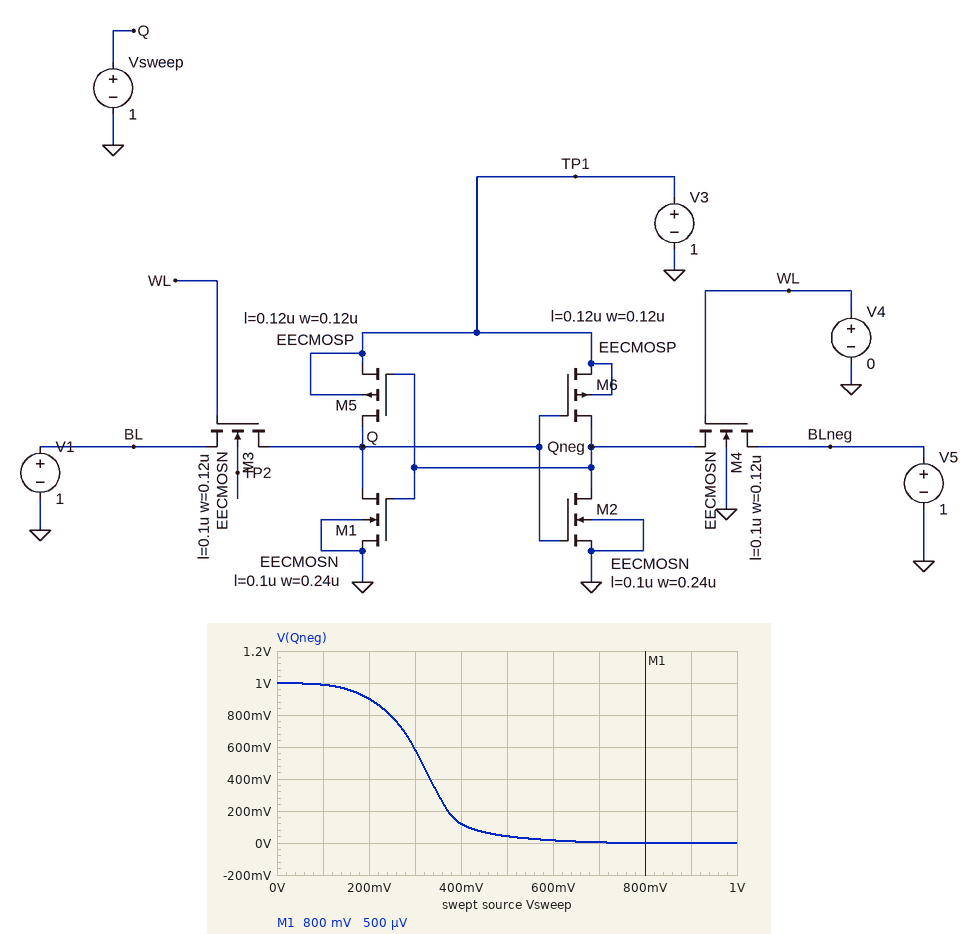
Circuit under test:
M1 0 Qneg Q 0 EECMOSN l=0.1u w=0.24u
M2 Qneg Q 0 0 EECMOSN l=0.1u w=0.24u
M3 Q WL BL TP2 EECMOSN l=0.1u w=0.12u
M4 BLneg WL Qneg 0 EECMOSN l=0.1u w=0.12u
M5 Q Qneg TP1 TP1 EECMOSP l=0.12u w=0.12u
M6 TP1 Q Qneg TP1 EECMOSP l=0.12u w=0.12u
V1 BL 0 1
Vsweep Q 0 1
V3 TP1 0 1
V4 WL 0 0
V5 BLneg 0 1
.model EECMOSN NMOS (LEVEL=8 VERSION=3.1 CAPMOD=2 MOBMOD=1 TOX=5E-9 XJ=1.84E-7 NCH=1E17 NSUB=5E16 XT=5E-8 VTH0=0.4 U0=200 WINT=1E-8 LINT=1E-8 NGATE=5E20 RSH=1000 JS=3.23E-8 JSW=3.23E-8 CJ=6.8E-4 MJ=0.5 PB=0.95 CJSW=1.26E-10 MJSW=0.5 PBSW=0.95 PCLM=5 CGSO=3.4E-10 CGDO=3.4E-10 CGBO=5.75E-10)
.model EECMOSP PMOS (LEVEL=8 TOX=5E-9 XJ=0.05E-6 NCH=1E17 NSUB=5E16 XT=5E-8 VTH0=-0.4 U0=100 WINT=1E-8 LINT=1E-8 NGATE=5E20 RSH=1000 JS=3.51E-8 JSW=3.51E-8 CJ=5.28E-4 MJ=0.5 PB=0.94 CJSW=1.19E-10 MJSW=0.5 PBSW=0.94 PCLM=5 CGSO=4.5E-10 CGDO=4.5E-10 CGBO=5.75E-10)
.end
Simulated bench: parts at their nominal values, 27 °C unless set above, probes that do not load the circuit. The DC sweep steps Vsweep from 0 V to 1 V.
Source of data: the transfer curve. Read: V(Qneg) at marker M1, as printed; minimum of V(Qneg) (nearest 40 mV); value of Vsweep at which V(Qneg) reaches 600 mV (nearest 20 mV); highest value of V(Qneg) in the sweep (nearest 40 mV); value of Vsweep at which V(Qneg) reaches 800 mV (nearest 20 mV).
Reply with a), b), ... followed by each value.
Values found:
a) 500 µV
b) 0 V
c) 300 mV
d) 1.00 V
e) 240 mV
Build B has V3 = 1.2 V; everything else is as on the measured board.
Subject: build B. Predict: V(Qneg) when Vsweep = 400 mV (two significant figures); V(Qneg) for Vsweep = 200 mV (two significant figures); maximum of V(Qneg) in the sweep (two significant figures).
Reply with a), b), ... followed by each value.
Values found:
a) 380 mV
b) 1.1 V
c) 1.2 V
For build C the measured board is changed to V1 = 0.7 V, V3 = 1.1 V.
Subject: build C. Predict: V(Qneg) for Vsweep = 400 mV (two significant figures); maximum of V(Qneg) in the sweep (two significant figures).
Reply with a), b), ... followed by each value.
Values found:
a) 230 mV
b) 1.1 V
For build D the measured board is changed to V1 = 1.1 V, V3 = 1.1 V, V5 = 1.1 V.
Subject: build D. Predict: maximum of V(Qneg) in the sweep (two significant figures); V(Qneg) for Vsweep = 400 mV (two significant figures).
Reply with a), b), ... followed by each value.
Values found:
a) 1.1 V
b) 230 mV
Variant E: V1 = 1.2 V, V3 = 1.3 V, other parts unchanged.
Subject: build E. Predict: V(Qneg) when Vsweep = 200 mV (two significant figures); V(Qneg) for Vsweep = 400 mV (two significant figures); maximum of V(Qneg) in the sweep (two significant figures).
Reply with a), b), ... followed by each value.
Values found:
a) 1.2 V
b) 520 mV
c) 1.3 V
